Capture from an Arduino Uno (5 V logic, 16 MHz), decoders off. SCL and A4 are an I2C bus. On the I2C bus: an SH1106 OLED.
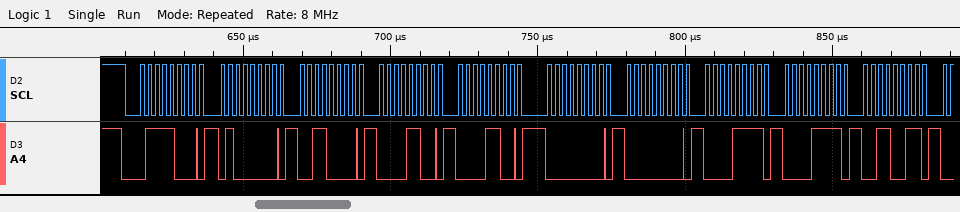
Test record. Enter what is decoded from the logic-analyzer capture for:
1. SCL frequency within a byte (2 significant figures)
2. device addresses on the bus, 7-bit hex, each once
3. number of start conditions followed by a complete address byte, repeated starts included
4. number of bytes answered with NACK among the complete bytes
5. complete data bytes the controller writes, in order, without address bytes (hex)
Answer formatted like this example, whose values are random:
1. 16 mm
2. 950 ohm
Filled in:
1. 400 kHz
2. 0x3C
3. 1
4. 0
5. 40 30 0C 0C 00 00 0F 0F 33
